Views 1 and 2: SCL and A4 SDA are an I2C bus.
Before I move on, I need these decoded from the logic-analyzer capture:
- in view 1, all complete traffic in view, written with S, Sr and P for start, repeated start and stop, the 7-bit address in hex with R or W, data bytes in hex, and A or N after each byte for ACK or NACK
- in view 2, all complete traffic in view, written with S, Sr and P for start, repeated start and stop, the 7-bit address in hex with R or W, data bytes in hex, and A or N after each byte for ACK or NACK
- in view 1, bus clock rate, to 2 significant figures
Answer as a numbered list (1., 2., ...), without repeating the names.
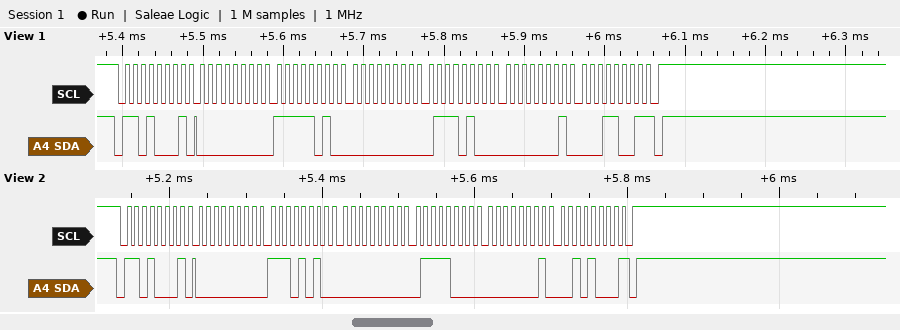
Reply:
1. S 68R A 00 A FA A 00 A 74 A 01 A 19 N P
2. S 68R A 00 A EA A 00 A 78 A 01 A 28 N P
3. 100 kHz
